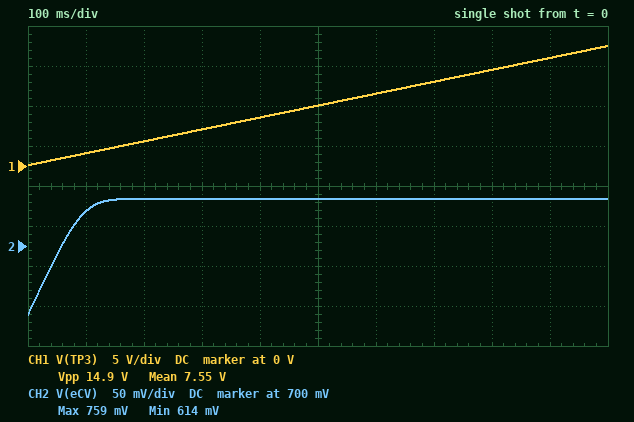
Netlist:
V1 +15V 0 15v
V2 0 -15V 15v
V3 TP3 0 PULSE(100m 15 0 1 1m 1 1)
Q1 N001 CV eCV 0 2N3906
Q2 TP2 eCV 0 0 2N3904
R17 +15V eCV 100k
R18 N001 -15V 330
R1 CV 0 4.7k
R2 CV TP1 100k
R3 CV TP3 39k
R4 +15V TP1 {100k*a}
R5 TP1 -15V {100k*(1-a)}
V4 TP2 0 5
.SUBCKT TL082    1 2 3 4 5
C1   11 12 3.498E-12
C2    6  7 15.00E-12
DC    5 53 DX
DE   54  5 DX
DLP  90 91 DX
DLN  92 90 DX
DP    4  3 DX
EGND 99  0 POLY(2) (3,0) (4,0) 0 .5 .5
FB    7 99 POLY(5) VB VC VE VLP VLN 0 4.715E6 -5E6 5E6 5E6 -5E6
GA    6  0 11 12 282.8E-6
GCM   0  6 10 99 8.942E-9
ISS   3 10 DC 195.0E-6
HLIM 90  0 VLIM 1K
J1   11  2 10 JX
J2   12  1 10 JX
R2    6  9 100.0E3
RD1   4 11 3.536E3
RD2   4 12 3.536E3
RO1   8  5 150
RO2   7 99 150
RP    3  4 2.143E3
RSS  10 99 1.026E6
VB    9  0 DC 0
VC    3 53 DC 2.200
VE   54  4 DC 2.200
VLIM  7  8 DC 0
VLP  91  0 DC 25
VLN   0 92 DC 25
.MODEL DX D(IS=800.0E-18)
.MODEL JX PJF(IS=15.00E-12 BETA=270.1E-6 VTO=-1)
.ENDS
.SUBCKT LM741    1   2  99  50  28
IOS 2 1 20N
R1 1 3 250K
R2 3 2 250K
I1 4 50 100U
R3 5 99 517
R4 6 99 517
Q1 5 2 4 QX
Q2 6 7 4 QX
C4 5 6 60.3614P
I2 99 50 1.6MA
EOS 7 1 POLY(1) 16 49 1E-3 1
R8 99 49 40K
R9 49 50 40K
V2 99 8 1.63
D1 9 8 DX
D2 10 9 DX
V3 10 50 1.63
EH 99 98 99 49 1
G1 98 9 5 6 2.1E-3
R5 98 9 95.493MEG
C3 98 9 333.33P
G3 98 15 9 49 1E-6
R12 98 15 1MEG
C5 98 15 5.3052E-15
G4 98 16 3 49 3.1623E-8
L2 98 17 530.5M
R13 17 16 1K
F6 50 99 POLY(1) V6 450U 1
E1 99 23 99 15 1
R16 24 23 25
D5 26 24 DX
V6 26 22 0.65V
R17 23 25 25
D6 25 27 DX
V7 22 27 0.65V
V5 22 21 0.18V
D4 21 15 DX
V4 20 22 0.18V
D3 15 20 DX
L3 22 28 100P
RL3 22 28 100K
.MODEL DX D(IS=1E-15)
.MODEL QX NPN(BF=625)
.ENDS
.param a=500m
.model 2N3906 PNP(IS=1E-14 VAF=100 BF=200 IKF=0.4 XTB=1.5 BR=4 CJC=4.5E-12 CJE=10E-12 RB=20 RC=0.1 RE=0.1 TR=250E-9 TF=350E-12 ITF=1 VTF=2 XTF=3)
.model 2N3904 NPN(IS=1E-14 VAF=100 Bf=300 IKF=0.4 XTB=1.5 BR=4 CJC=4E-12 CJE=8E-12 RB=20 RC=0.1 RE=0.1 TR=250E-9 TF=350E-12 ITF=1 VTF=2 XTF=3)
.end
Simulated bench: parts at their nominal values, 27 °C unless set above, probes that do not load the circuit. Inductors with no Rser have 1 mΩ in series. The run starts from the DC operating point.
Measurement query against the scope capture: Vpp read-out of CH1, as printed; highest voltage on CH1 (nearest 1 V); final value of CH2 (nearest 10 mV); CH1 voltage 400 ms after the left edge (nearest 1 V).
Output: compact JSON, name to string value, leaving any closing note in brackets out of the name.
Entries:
{"Vpp read-out of CH1, as printed": "14.9 V", "highest voltage on CH1": "15 V", "final value of CH2": "760 mV", "CH1 voltage 400 ms after the left edge": "6 V"}
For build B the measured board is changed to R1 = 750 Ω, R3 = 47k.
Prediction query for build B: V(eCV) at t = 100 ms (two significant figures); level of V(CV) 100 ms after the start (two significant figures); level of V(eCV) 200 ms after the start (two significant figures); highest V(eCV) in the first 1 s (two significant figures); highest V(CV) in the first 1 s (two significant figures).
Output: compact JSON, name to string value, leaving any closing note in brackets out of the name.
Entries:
{"V(eCV) at t = 100 ms": "630 mV", "level of V(CV) 100 ms after the start": "25 mV", "level of V(eCV) 200 ms after the start": "650 mV", "highest V(eCV) in the first 1 s": "760 mV", "highest V(CV) in the first 1 s": "230 mV"}
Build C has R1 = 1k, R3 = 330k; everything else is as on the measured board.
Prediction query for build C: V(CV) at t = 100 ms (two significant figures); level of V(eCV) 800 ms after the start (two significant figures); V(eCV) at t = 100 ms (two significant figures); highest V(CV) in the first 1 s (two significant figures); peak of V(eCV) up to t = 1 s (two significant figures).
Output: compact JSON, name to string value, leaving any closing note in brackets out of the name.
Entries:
{"V(CV) at t = 100 ms": "5.4 mV", "level of V(eCV) 800 ms after the start": "640 mV", "V(eCV) at t = 100 ms": "610 mV", "highest V(CV) in the first 1 s": "46 mV", "peak of V(eCV) up to t = 1 s": "650 mV"}
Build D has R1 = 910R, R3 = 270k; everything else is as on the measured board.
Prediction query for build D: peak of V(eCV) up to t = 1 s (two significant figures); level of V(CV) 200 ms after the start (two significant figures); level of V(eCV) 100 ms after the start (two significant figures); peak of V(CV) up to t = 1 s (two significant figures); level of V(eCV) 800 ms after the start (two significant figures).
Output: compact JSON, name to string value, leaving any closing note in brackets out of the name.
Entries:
{"peak of V(eCV) up to t = 1 s": "650 mV", "level of V(CV) 200 ms after the start": "11 mV", "level of V(eCV) 100 ms after the start": "610 mV", "peak of V(CV) up to t = 1 s": "51 mV", "level of V(eCV) 800 ms after the start": "640 mV"}
